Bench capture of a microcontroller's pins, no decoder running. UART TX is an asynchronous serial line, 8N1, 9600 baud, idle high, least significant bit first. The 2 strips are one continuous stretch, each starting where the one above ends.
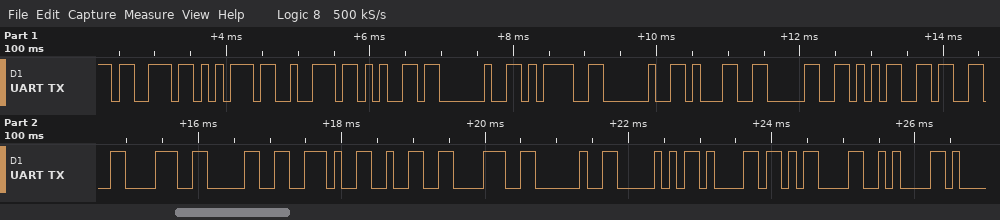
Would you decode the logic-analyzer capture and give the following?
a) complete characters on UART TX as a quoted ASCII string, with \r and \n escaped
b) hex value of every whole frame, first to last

"sure = 105380.28 Pa\r\n"
73 75 72 65 20 3D 20 31 30 35 33 38 30 2E 32 38 20 50 61 0D 0A
